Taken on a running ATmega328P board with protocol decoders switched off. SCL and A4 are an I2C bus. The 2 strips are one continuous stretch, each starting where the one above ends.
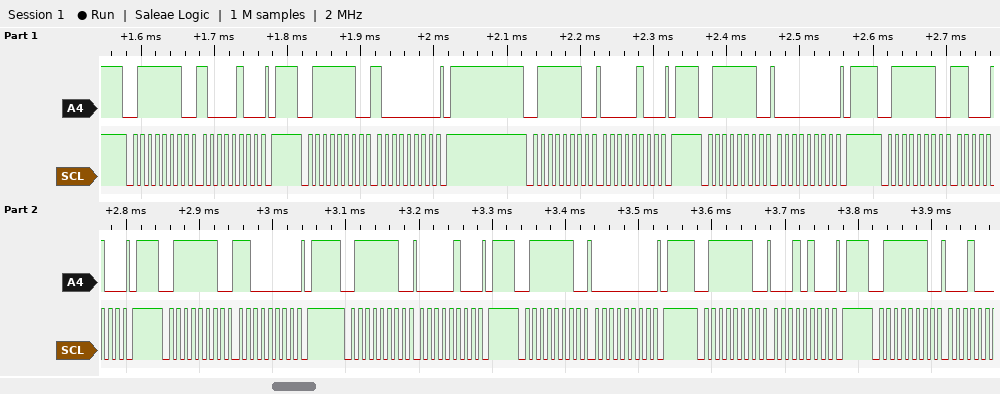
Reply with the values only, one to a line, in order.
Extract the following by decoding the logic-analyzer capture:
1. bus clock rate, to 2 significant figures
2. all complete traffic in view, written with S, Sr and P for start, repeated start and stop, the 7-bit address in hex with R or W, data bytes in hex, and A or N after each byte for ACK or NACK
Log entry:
100 kHz
S 3FW A 84 A P S 3FW A 80 A P S 3FW A 04 A P S 3FW A 00 A P S 3FW A C4 A P S 3FW A C0 A P S 3FW A 04 A P S 3FW A 00 A P S 3FW A 14 A P S 3FW A
